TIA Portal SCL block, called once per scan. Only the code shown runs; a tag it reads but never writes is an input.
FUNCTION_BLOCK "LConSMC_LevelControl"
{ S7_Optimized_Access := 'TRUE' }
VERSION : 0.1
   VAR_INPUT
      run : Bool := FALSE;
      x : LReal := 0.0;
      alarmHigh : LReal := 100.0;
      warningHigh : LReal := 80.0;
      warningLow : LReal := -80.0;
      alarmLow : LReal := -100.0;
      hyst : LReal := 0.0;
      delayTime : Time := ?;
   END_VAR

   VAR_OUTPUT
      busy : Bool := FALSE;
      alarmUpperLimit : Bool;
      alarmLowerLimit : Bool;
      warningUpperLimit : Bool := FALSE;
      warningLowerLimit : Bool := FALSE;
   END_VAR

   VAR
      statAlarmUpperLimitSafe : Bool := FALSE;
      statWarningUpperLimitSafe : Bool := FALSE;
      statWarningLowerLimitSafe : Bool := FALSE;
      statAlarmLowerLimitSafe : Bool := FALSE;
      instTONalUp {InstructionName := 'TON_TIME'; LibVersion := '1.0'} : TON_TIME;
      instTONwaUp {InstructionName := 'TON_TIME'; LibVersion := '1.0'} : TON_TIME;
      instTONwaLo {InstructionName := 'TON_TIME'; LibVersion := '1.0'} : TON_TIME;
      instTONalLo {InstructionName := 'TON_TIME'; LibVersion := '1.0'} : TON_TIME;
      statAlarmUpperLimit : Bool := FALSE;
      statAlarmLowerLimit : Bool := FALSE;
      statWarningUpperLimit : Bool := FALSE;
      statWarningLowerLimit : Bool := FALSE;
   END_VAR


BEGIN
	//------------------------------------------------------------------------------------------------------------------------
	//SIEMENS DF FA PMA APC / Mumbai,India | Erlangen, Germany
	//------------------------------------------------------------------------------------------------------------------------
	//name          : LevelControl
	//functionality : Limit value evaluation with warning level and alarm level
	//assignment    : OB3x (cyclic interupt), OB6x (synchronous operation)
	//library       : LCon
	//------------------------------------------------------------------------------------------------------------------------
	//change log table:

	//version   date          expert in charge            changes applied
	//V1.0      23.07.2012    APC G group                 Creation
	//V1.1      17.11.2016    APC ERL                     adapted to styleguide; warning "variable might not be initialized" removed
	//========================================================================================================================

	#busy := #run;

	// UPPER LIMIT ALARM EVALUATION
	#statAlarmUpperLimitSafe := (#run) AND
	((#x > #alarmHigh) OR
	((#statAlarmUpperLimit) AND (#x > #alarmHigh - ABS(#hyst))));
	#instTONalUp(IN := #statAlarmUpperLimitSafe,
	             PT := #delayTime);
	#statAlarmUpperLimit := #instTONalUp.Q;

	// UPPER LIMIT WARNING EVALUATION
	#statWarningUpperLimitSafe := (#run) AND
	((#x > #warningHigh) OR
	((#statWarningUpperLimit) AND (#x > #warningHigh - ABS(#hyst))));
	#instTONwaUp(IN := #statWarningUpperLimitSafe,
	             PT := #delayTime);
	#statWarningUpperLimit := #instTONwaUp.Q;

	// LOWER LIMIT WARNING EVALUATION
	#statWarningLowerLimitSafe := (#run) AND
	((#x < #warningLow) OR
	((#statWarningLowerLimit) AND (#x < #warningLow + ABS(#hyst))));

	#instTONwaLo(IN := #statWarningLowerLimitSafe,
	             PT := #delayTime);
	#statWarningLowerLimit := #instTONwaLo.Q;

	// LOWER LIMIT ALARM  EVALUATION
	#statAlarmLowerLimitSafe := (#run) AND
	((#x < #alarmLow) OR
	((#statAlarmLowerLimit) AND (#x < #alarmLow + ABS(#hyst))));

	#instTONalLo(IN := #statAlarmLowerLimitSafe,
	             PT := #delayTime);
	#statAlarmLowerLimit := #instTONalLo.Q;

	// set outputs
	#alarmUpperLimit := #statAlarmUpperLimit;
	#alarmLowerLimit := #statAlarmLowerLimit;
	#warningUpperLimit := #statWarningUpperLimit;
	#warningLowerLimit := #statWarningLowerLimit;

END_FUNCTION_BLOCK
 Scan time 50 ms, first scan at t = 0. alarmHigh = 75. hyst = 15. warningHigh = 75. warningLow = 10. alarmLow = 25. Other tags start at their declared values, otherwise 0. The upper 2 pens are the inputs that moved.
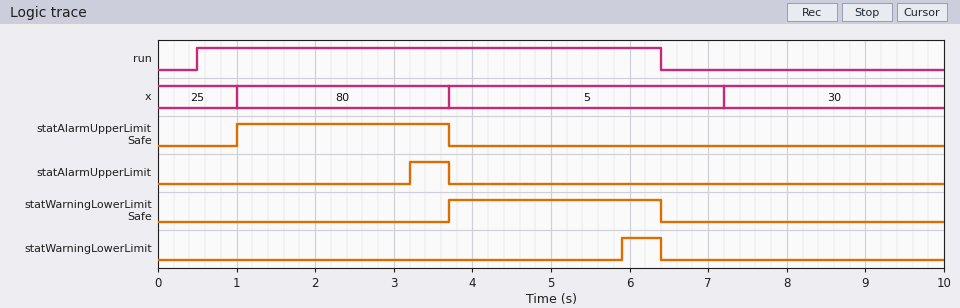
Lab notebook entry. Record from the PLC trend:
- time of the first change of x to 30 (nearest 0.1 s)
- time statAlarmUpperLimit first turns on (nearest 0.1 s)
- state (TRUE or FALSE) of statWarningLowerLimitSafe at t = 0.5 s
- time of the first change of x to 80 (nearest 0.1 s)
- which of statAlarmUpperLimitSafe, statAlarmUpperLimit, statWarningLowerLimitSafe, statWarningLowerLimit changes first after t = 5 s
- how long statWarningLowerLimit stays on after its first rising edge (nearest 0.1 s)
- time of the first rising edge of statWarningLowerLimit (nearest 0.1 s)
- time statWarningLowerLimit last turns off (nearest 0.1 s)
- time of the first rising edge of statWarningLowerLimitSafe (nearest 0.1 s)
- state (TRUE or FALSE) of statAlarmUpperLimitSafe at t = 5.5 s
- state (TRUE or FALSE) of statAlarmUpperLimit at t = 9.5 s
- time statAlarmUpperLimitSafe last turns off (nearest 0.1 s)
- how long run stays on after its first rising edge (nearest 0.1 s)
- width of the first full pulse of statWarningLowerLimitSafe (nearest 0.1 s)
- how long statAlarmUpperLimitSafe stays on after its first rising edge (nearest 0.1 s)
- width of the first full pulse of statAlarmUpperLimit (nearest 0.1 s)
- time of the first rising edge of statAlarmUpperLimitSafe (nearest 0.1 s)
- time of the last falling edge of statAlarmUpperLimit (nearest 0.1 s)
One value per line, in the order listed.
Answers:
7.2 s
3.2 s
FALSE
1.0 s
statWarningLowerLimit
0.5 s
5.9 s
6.4 s
3.7 s
FALSE
FALSE
3.7 s
5.9 s
2.7 s
2.7 s
0.5 s
1.0 s
3.7 s
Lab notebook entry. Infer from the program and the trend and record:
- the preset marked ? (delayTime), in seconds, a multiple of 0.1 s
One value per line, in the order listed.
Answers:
2.2 s
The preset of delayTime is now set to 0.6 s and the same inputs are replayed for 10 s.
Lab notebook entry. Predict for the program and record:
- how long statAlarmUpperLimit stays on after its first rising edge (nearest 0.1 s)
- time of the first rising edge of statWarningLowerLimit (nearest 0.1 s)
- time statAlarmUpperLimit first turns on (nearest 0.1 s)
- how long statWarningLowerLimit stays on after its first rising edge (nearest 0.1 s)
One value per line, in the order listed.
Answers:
2.1 s
4.3 s
1.6 s
2.1 s
